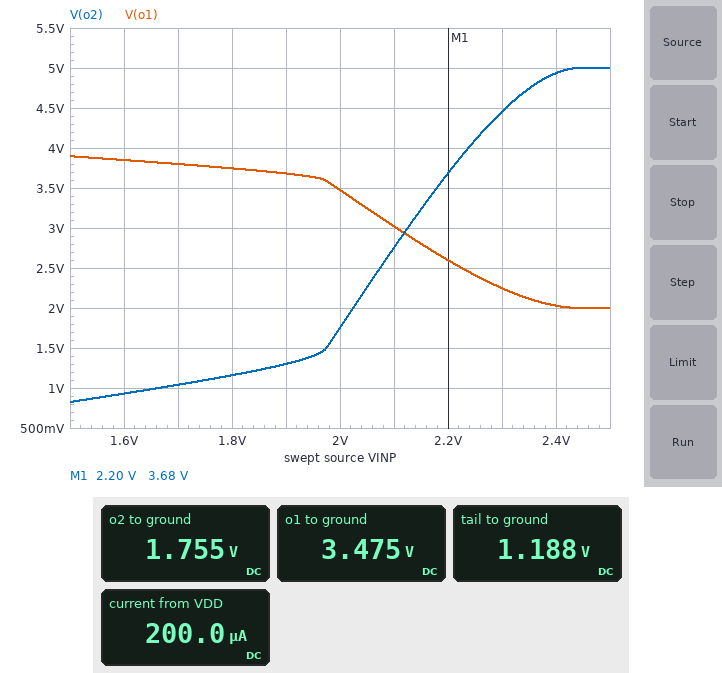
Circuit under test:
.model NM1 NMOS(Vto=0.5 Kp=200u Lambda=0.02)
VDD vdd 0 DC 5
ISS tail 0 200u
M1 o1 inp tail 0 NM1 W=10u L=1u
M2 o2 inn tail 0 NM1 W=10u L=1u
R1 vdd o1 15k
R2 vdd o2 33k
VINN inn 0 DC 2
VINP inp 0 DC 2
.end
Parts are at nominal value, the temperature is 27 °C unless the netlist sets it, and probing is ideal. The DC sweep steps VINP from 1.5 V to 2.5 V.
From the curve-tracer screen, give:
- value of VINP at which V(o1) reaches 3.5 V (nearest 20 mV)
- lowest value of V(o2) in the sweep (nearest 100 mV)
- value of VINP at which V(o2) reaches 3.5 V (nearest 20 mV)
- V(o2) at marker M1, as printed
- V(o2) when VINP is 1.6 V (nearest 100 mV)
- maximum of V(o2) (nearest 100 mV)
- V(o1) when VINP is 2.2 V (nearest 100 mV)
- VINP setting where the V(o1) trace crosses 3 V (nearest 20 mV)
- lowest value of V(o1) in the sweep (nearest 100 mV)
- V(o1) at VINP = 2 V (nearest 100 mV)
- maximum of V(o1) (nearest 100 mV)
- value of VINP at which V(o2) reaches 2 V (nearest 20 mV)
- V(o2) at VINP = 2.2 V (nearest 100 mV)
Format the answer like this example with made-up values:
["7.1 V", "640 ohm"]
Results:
["2.00 V", "800 mV", "2.18 V", "3.68 V", "900 mV", "5.0 V", "2.6 V", "2.10 V", "2.0 V", "3.5 V", "3.9 V", "2.02 V", "3.7 V"]
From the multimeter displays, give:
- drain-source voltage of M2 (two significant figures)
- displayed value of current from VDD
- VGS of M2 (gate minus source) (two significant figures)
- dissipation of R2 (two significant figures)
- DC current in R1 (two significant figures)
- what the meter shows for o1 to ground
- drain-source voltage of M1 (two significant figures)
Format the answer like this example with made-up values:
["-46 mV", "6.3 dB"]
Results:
["570 mV", "200.0 µA", "810 mV", "320 µW", "100 µA", "3.475 V", "2.3 V"]
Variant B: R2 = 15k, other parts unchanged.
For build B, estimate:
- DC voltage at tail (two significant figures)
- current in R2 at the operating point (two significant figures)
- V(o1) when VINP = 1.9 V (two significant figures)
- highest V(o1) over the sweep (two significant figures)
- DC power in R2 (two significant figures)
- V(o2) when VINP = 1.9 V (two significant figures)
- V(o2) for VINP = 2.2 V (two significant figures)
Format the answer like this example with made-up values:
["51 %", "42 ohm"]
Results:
["1.2 V", "100 µA", "4.0 V", "5.0 V", "150 µW", "3.0 V", "4.4 V"]
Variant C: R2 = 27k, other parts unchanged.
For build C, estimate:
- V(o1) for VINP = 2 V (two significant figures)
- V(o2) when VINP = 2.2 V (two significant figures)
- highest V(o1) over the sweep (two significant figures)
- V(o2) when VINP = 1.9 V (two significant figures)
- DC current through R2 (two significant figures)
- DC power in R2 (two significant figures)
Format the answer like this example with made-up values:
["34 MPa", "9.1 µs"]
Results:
["3.5 V", "3.9 V", "4.3 V", "1.5 V", "99 µA", "260 µW"]
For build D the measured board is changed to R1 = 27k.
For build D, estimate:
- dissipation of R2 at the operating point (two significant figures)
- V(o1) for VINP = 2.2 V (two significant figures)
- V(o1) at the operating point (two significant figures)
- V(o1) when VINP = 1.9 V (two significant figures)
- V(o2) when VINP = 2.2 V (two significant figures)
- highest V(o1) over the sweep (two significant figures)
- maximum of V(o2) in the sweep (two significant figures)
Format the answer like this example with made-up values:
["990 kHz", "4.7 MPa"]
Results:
["330 µW", "1.4 V", "2.3 V", "2.6 V", "2.8 V", "3.0 V", "2.9 V"]
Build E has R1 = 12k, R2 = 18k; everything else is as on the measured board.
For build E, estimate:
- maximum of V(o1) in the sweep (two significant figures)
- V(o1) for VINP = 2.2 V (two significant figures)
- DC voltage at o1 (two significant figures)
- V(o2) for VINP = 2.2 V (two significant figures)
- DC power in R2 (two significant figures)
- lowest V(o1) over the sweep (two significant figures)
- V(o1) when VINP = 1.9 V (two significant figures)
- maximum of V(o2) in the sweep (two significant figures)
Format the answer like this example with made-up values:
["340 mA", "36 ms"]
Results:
["5.0 V", "3.1 V", "3.8 V", "4.3 V", "180 µW", "2.6 V", "4.2 V", "5.0 V"]
